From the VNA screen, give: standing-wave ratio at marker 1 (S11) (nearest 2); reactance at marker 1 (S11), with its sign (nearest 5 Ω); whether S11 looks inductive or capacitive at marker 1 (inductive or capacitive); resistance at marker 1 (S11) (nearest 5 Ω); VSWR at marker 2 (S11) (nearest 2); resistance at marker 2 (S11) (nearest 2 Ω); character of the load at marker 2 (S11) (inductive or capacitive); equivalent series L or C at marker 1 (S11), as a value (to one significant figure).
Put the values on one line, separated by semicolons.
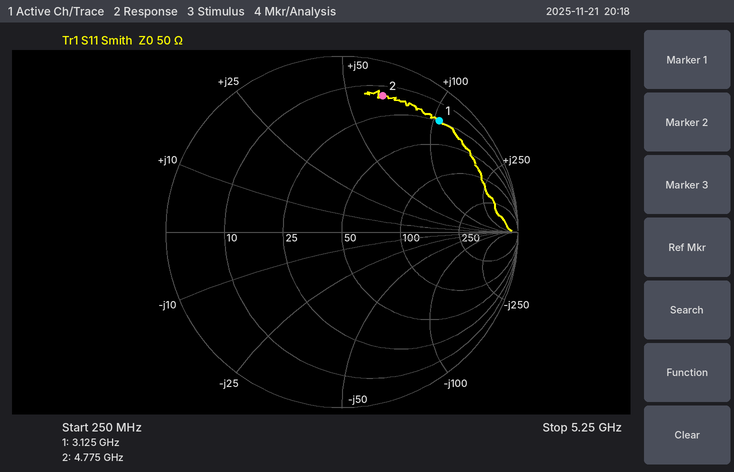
12; +105 Ω; inductive; 25 Ω; 10; 14 Ω; inductive; 5 nH
